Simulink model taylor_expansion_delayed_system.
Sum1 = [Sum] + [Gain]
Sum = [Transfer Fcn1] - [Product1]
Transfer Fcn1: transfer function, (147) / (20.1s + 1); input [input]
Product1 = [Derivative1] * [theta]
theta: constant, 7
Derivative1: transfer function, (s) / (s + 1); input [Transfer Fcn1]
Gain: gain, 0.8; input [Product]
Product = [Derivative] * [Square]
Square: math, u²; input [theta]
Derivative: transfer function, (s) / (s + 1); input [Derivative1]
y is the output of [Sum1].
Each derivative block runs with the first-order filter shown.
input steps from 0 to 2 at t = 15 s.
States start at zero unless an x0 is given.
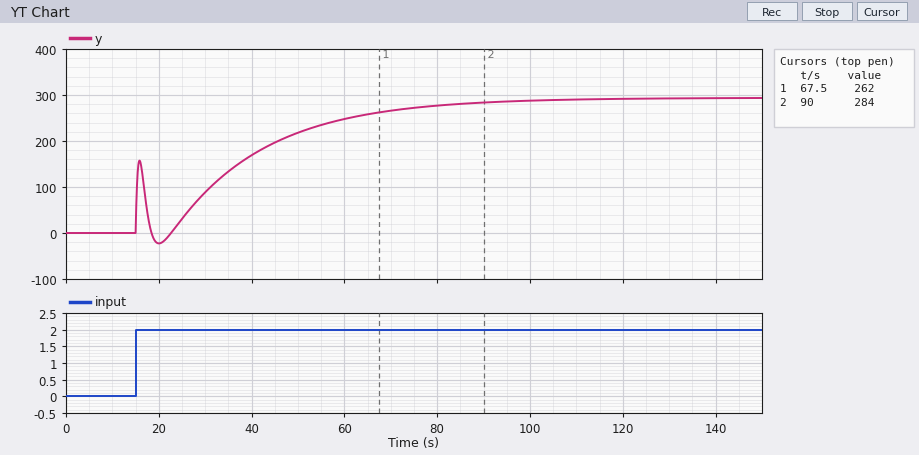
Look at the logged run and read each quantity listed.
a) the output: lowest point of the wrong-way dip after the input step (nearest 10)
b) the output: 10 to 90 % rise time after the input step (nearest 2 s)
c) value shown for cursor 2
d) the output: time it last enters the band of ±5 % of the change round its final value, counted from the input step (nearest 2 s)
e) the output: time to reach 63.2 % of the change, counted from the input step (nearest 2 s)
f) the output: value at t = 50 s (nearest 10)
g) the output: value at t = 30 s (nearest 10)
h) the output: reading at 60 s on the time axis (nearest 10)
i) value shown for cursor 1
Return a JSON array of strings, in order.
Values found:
["-20", "54 s", "284", "68 s", "28 s", "220", "90", "250", "262"]
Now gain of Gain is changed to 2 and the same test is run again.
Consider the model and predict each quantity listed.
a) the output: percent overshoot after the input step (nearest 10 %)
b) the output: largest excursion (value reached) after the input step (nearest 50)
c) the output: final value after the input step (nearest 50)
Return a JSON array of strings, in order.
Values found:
["60 %", "450", "300"]
